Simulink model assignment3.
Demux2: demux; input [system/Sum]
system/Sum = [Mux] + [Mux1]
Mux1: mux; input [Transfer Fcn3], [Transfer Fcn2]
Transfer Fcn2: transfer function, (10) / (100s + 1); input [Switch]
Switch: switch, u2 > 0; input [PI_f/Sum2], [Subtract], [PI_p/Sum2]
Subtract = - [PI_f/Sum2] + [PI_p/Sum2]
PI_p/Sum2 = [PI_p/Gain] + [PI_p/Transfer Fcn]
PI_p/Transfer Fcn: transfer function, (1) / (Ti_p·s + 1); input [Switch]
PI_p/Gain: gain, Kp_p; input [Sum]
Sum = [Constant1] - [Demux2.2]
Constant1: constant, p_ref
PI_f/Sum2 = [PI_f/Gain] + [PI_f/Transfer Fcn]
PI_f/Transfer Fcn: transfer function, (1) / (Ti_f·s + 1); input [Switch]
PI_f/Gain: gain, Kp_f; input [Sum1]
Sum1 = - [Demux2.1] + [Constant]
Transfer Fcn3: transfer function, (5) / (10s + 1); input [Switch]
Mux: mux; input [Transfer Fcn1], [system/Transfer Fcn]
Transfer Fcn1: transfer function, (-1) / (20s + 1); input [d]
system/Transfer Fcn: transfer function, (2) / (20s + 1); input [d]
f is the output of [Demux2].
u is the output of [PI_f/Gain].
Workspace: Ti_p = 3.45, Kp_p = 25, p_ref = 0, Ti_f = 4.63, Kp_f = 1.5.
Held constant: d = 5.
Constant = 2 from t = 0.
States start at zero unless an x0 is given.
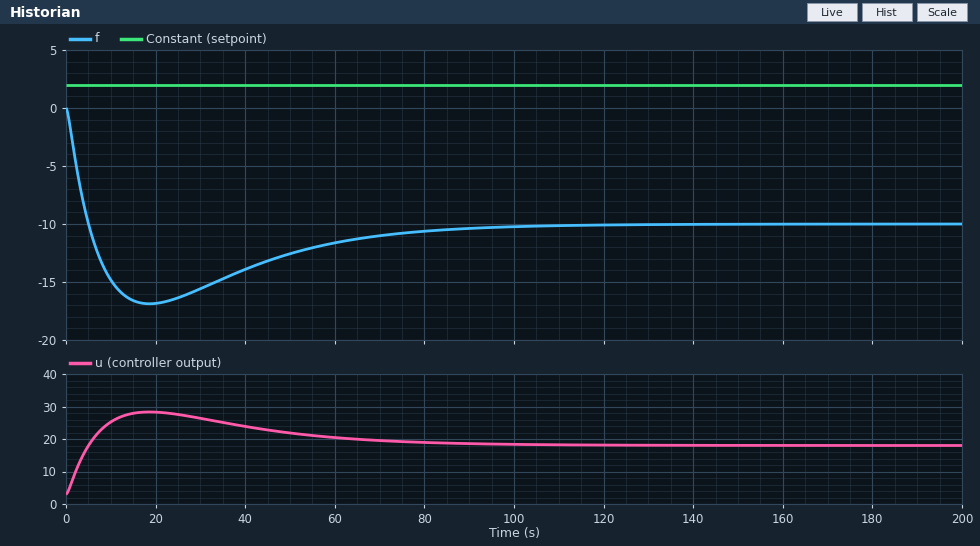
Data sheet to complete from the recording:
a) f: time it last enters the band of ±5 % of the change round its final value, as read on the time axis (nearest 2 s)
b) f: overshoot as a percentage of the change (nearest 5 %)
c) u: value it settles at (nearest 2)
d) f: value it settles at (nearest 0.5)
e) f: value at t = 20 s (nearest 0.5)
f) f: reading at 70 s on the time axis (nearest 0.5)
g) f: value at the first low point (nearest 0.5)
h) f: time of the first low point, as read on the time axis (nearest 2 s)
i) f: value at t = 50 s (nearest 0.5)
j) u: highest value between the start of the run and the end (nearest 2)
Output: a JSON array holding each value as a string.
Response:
["84 s", "70 %", "18", "-10.0", "-17.0", "-11.0", "-17.0", "18 s", "-12.5", "28"]
